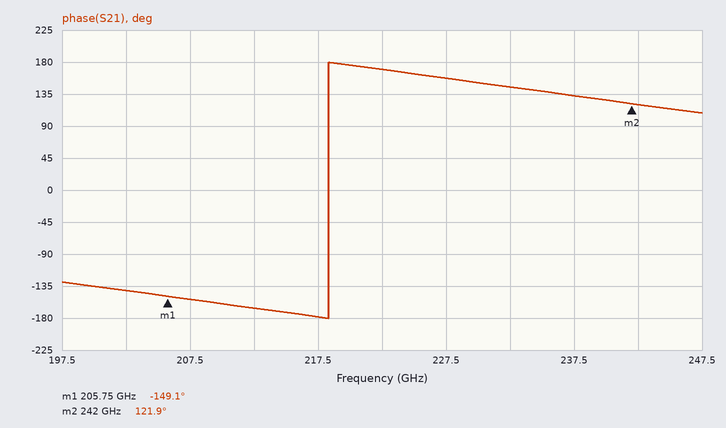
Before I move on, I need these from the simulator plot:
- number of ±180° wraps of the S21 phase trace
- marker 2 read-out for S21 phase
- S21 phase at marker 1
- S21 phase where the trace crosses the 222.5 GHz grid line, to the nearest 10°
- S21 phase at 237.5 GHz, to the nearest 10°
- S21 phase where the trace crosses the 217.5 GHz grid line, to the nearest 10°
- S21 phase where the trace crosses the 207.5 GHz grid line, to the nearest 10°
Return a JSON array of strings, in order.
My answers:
["1", "121.9°", "-149.1°", "170°", "130°", "-180°", "-150°"]
